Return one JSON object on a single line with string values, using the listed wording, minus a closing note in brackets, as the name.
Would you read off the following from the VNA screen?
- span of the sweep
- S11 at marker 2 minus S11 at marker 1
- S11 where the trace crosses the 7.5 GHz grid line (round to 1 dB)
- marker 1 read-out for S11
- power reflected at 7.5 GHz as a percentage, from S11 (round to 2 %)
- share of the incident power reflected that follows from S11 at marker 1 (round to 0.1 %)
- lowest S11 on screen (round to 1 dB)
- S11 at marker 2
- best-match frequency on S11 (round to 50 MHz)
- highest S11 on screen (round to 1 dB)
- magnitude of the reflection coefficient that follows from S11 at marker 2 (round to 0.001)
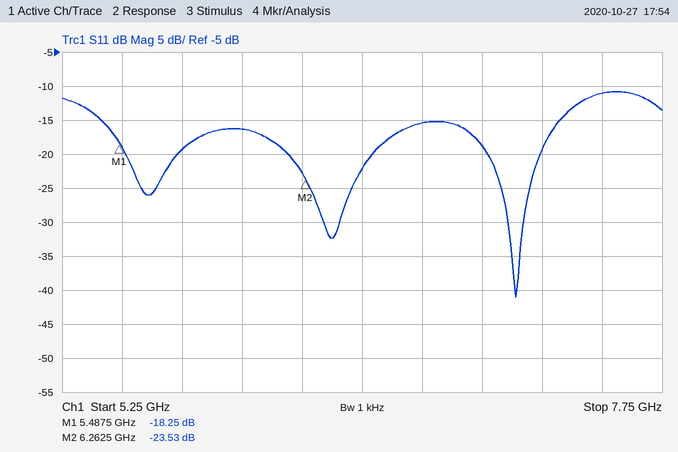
{"span of the sweep": "2.5 GHz", "S11 at marker 2 minus S11 at marker 1": "-5.28 dB", "S11 where the trace crosses the 7.5 GHz grid line": "-11 dB", "marker 1 read-out for S11": "-18.25 dB", "power reflected at 7.5 GHz as a percentage, from S11": "8 %", "share of the incident power reflected that follows from S11 at marker 1": "1.5 %", "lowest S11 on screen": "-41 dB", "S11 at marker 2": "-23.53 dB", "best-match frequency on S11": "7.15 GHz", "highest S11 on screen": "-11 dB", "magnitude of the reflection coefficient that follows from S11 at marker 2": "0.067"}
